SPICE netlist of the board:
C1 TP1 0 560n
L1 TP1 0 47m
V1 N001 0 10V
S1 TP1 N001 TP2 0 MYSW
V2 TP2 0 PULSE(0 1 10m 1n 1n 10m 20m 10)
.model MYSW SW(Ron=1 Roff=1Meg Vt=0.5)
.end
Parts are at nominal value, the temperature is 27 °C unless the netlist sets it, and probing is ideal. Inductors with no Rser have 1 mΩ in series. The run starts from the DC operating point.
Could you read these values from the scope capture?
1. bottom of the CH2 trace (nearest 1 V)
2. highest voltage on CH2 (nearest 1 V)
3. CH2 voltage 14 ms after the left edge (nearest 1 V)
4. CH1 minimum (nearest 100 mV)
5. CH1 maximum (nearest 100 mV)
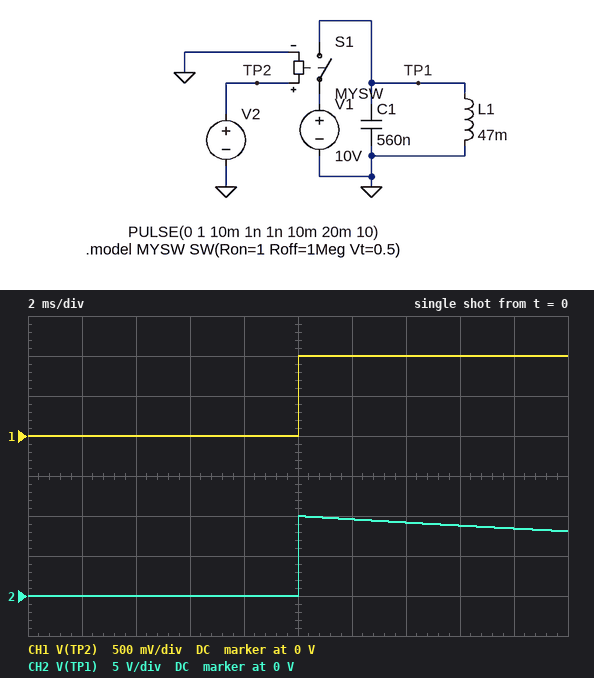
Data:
0 V
10 V
9 V
0 V
1.0 V
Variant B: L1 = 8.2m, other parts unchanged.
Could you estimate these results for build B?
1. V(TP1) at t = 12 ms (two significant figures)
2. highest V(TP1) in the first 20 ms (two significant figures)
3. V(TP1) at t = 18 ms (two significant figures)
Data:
7.8 V
10 V
3.8 V
